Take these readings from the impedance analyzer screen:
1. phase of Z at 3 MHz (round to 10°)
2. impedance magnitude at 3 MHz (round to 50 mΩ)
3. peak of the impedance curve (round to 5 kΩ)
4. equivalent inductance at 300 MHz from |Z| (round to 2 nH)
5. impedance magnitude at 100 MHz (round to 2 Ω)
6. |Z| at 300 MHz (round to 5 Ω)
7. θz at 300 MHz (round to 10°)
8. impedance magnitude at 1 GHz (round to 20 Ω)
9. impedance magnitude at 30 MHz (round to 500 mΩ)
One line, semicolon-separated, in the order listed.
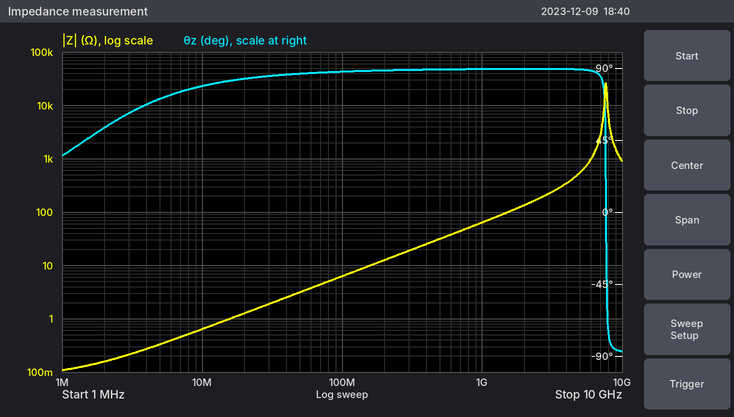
60°; 200 mΩ; 25 kΩ; 10 nH; 6 Ω; 20 Ω; 90°; 60 Ω; 2.0 Ω
